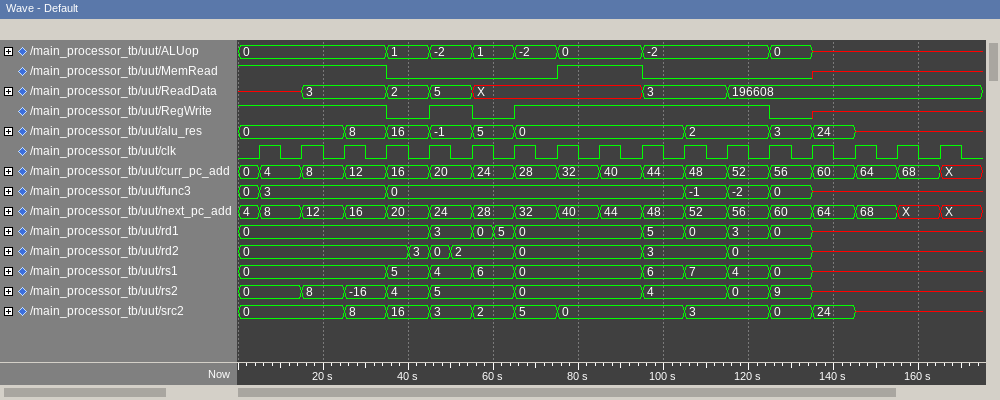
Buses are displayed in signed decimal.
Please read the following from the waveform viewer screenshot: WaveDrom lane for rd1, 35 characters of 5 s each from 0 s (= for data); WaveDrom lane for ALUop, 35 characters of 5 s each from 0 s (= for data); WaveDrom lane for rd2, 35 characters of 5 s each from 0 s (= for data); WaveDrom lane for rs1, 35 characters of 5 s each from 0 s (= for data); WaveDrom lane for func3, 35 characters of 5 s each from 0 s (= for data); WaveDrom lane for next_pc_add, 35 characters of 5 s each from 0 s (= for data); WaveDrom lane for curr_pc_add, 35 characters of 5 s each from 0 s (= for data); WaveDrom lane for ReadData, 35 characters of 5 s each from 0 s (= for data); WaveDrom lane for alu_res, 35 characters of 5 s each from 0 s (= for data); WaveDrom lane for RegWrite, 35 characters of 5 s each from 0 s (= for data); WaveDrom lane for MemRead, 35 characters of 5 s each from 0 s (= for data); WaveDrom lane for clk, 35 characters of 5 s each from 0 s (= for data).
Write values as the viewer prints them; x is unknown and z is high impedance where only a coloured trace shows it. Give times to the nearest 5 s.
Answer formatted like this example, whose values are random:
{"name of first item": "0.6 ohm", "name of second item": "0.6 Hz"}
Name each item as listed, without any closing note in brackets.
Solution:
{"WaveDrom lane for rd1, 35 characters of 5 s each from 0 s": "{name: 'rd1', wave: '=........=.===.....=.=.=.=.x.......', data: '0 3 0 5 0 5 0 3 0'}", "WaveDrom lane for ALUop, 35 characters of 5 s each from 0 s": "{name: 'ALUop', wave: '=......=.=.=.=.=...=.....=.x.......', data: '0 1 -2 1 -2 0 -2 0'}", "WaveDrom lane for rd2, 35 characters of 5 s each from 0 s": "{name: 'rd2', wave: '=.......===..=.....=...=...x.......', data: '0 3 0 2 0 3 0'}", "WaveDrom lane for rs1, 35 characters of 5 s each from 0 s": "{name: 'rs1', wave: '=......=.=.=.=.....=.=.=.=.x.......', data: '0 5 4 6 0 6 7 4 0'}", "WaveDrom lane for func3, 35 characters of 5 s each from 0 s": "{name: 'func3', wave: '==.....=.............=.=.=.x.......', data: '0 3 0 -1 -2 0'}", "WaveDrom lane for next_pc_add, 35 characters of 5 s each from 0 s": "{name: 'next_pc_add', wave: '==.=.=.=.=.=.=.=.=.=.=.=.=.=.=.=.=.', data: '4 8 12 16 20 24 28 32 40 44 48 52 56 60 64 68 X X'}", "WaveDrom lane for curr_pc_add, 35 characters of 5 s each from 0 s": "{name: 'curr_pc_add', wave: '==.=.=.=.=.=.=.=.=.=.=.=.=.=.=.=.=.', data: '0 4 8 12 16 20 24 28 32 40 44 48 52 56 60 64 68 X'}", "WaveDrom lane for ReadData, 35 characters of 5 s each from 0 s": "{name: 'ReadData', wave: 'x..=...=.=.=.......=...=...........', data: '3 2 5 X 3 196608'}", "WaveDrom lane for alu_res, 35 characters of 5 s each from 0 s": "{name: 'alu_res', wave: '=....=.=.=.=.=.......=...=.=.x.....', data: '0 8 16 -1 5 0 2 3 24'}", "WaveDrom lane for RegWrite, 35 characters of 5 s each from 0 s": "{name: 'RegWrite', wave: '1......0.1.0.1...........0.x.......'}", "WaveDrom lane for MemRead, 35 characters of 5 s each from 0 s": "{name: 'MemRead', wave: '1......0.......1...0.......x.......'}", "WaveDrom lane for clk, 35 characters of 5 s each from 0 s": "{name: 'clk', wave: '01010101010101010101010101010101010'}"}
